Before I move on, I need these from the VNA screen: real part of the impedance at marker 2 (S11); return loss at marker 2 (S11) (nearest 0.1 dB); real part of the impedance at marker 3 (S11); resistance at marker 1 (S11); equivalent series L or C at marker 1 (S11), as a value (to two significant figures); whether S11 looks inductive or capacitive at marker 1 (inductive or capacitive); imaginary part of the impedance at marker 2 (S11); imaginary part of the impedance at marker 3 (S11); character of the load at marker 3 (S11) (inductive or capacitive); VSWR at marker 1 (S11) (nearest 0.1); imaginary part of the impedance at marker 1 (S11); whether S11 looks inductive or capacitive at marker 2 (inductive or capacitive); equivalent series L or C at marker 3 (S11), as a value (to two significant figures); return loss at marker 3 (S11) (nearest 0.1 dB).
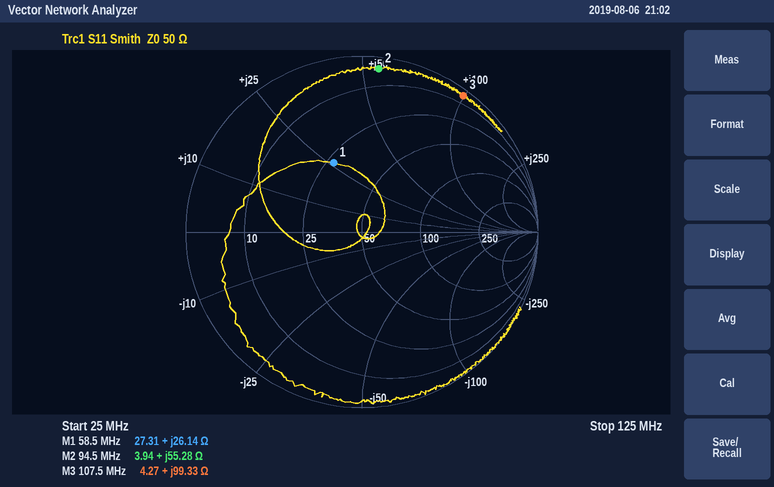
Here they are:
3.94 Ω
0.6 dB
4.27 Ω
27.31 Ω
71 nH
inductive
+55.28 Ω
+99.33 Ω
inductive
2.5
+26.14 Ω
inductive
150 nH
0.3 dB
